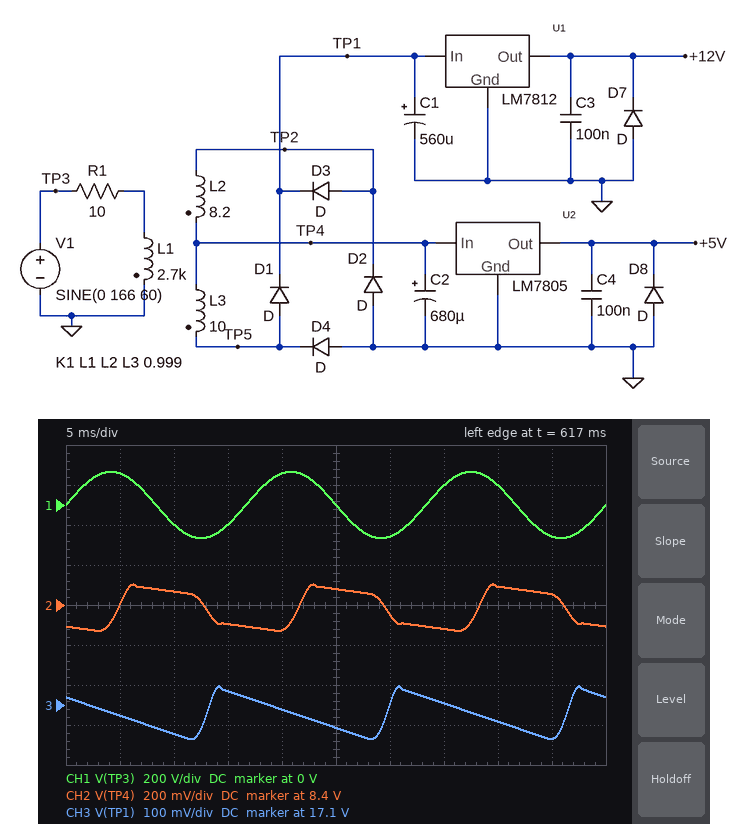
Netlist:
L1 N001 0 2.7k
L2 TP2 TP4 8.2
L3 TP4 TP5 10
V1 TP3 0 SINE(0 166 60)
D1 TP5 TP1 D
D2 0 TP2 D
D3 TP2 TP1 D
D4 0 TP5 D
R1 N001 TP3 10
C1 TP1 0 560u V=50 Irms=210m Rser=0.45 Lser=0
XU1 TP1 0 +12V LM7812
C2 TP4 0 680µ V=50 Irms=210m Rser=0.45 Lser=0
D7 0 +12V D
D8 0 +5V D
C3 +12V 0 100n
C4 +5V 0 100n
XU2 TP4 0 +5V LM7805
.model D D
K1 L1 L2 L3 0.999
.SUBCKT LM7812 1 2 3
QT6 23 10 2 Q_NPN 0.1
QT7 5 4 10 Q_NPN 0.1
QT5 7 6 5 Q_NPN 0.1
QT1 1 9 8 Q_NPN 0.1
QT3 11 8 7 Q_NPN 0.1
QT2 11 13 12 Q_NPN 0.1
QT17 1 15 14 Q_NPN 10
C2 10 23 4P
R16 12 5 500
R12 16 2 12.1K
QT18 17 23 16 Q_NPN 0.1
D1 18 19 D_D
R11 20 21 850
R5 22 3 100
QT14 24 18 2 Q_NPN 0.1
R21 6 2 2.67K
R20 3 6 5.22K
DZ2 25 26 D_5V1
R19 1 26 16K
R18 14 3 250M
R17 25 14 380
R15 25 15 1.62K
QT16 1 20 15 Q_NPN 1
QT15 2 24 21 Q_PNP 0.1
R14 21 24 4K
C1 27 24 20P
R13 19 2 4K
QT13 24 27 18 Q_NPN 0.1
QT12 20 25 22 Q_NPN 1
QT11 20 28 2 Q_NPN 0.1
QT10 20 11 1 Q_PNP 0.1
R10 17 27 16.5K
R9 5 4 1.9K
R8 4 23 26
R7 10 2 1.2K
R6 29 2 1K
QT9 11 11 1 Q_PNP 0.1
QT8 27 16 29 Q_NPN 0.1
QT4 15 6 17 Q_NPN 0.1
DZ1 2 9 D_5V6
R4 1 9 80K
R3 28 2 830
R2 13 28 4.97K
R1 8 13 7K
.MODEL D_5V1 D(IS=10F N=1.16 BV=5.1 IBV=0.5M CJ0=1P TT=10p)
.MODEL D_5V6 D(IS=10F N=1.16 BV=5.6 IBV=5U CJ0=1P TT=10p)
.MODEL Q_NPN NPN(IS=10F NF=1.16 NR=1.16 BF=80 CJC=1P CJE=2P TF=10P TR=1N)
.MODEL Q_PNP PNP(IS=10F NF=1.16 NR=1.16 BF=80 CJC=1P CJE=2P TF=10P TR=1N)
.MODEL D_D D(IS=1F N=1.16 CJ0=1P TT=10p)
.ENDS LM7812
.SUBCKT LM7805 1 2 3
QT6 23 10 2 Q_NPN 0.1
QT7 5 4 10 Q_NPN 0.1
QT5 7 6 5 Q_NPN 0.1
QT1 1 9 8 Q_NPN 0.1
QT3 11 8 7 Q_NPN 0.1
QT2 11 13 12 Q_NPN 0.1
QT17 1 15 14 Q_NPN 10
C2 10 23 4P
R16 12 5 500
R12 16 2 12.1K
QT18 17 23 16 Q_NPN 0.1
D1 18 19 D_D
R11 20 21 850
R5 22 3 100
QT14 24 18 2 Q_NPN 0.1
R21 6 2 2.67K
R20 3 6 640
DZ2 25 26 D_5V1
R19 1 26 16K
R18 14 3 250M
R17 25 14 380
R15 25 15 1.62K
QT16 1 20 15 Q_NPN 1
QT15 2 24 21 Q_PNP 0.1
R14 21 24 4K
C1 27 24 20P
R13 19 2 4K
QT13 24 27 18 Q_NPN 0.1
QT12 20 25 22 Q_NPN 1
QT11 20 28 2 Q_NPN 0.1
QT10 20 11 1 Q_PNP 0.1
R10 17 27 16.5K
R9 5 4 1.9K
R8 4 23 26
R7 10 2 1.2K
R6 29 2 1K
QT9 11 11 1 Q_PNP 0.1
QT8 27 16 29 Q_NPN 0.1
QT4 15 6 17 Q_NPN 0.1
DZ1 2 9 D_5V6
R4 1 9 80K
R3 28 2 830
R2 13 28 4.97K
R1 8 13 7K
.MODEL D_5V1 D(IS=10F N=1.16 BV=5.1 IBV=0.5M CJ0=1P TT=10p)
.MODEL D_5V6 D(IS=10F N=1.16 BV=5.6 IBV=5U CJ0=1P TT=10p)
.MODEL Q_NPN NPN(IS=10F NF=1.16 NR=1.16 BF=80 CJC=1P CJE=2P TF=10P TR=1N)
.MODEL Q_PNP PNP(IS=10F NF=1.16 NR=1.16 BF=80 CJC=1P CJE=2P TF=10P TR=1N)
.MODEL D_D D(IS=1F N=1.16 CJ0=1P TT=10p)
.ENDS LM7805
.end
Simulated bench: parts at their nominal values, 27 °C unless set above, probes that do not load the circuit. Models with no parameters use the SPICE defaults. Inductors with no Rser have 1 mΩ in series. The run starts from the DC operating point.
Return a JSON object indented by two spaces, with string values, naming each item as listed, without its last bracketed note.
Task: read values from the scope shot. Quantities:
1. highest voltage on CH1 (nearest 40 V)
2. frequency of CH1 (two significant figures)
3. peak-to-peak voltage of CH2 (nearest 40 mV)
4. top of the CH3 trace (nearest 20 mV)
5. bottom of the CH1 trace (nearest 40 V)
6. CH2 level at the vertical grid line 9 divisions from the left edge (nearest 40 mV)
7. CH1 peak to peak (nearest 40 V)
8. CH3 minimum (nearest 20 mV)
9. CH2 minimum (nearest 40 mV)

{
  "highest voltage on CH1": "160 V",
  "frequency of CH1": "60 Hz",
  "peak-to-peak voltage of CH2": "240 mV",
  "top of the CH3 trace": "17.14 V",
  "bottom of the CH1 trace": "-160 V",
  "CH2 level at the vertical grid line 9 divisions from the left edge": "8.44 V",
  "CH1 peak to peak": "320 V",
  "CH3 minimum": "17.02 V",
  "CH2 minimum": "8.28 V"
}
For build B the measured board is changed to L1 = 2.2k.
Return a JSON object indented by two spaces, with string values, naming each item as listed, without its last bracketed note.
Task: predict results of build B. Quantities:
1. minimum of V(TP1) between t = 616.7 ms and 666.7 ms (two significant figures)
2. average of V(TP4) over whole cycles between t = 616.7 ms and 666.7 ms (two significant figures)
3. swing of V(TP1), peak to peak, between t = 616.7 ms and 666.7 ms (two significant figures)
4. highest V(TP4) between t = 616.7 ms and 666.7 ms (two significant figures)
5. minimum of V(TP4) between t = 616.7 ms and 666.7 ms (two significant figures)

{
  "minimum of V(TP1) between t = 616.7 ms and 666.7 ms": "19 V",
  "average of V(TP4) over whole cycles between t = 616.7 ms and 666.7 ms": "9.4 V",
  "swing of V(TP1), peak to peak, between t = 616.7 ms and 666.7 ms": "130 mV",
  "highest V(TP4) between t = 616.7 ms and 666.7 ms": "9.5 V",
  "minimum of V(TP4) between t = 616.7 ms and 666.7 ms": "9.3 V"
}
